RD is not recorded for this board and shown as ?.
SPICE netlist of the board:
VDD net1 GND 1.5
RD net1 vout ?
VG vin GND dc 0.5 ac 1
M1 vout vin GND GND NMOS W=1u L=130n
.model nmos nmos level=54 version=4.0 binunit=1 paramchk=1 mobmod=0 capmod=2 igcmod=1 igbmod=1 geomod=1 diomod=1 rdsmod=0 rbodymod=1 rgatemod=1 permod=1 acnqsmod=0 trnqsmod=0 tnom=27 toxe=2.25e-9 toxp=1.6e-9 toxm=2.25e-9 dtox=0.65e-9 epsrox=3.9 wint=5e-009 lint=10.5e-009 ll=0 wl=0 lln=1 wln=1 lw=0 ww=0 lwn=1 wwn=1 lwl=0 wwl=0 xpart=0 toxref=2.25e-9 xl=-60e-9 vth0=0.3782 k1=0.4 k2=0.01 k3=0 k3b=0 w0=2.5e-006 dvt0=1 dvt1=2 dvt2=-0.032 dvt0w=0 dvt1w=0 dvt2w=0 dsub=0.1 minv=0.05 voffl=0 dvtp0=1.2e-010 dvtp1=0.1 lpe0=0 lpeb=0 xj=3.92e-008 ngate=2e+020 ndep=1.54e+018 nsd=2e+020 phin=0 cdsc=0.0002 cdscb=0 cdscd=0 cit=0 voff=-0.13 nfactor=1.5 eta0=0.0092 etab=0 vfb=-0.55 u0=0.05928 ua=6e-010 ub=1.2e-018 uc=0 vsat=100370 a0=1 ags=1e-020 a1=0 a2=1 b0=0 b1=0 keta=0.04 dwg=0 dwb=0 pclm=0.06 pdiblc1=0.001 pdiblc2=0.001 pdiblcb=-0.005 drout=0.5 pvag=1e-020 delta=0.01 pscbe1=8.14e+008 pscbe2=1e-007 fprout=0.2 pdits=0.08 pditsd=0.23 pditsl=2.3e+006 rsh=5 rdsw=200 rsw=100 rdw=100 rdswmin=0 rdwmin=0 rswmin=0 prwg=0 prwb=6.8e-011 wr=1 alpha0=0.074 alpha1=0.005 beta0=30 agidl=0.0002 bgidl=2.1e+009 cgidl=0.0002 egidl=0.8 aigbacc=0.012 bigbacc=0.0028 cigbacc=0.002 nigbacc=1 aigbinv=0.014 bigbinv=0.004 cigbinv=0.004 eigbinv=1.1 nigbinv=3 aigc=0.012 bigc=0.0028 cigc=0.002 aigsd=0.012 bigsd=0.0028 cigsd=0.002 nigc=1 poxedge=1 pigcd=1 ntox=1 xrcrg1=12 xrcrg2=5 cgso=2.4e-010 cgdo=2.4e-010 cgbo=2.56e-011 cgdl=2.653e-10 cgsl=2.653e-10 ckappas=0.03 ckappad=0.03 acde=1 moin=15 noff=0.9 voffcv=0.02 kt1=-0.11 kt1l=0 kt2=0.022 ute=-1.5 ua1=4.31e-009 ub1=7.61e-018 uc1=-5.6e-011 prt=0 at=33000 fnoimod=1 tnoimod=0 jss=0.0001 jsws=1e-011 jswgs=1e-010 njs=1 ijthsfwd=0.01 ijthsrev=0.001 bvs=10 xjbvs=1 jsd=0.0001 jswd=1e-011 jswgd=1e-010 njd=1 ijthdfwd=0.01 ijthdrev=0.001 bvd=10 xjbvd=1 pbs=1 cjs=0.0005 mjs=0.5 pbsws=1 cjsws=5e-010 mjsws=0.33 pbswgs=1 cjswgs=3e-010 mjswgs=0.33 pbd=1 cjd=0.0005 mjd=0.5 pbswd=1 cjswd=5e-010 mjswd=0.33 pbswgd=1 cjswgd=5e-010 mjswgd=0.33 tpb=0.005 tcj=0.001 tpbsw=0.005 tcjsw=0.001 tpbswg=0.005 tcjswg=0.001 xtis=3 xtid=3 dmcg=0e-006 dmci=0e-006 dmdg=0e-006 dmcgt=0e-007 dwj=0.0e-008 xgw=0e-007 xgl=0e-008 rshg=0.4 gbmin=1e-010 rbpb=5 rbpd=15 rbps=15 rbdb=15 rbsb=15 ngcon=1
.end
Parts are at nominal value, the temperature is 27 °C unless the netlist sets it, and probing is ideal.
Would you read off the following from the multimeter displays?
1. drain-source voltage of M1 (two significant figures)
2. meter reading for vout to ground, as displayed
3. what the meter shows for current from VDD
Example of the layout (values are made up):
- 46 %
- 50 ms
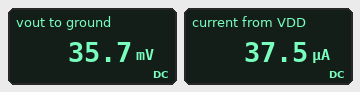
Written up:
- 36 mV
- 35.7 mV
- 37.5 µA
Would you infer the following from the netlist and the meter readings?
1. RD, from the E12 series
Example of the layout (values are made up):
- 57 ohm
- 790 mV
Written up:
- 39 kΩ
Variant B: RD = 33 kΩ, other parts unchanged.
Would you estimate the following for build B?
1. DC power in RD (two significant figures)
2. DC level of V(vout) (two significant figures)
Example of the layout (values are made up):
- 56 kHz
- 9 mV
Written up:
- 64 µW
- 44 mV
